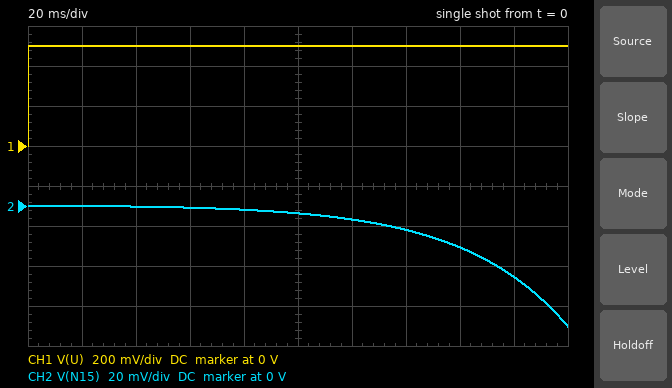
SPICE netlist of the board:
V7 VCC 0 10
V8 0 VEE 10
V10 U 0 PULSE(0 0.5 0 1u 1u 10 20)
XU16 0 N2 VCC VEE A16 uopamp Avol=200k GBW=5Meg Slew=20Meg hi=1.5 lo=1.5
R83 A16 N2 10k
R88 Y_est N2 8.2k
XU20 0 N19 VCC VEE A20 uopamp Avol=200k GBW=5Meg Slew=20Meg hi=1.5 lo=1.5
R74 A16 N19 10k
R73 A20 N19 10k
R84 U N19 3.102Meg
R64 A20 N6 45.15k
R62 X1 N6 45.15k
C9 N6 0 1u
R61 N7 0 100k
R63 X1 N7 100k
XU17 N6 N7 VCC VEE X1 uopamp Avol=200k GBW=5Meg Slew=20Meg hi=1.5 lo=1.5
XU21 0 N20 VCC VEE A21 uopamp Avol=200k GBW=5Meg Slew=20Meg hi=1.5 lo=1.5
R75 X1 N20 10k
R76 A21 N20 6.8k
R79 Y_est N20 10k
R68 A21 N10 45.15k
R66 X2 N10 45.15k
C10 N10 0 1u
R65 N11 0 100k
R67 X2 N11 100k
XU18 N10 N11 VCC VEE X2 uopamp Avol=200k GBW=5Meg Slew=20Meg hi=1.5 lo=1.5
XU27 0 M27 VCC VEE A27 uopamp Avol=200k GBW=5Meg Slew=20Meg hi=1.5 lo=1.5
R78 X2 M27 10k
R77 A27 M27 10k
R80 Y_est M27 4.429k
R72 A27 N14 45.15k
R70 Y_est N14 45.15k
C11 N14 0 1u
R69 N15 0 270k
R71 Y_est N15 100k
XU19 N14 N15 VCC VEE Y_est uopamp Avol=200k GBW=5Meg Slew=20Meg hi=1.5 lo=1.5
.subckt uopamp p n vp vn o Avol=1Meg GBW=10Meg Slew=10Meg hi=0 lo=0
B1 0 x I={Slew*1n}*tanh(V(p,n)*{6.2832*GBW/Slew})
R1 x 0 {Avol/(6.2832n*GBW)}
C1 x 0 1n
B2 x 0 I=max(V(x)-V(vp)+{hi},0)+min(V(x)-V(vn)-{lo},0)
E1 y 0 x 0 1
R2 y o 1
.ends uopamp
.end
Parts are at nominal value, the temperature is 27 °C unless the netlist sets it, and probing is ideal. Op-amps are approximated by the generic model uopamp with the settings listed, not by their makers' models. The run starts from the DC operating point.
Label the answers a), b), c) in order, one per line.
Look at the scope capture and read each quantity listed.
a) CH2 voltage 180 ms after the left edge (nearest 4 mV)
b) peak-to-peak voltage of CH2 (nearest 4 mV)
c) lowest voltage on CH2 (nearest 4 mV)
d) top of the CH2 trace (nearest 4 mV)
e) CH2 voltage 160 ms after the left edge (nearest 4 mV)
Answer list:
a) -36 mV
b) 60 mV
c) -60 mV
d) 0 V
e) -20 mV
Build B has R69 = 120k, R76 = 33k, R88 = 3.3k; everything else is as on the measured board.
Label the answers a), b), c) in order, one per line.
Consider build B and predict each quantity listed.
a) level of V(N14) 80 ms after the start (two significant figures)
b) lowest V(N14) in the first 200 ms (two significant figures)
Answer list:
a) -76 mV
b) -2.0 V
